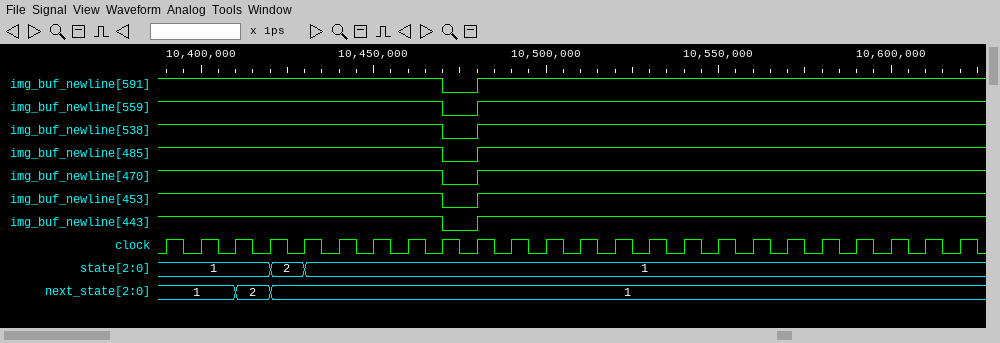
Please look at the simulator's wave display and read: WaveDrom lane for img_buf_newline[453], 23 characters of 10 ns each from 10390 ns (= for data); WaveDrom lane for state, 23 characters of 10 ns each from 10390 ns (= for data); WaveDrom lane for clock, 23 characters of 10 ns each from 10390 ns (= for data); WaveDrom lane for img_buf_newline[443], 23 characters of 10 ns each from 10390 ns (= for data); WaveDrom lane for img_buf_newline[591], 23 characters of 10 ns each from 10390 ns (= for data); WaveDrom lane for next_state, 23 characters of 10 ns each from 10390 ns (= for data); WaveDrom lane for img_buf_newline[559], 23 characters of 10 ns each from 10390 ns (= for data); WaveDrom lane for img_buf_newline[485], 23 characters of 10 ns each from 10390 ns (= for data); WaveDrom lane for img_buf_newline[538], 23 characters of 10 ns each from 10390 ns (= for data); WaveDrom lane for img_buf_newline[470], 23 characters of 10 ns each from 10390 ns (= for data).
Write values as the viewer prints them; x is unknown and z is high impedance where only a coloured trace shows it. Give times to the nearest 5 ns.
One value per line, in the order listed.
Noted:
{name: 'img_buf_newline[453]', wave: '1.......01.............'}
{name: 'state', wave: '=..==..................', data: '1 2 1'}
{name: 'clock', wave: 'p......................'}
{name: 'img_buf_newline[443]', wave: '1.......01.............'}
{name: 'img_buf_newline[591]', wave: '1.......01.............'}
{name: 'next_state', wave: '=.==...................', data: '1 2 1'}
{name: 'img_buf_newline[559]', wave: '1.......01.............'}
{name: 'img_buf_newline[485]', wave: '1.......01.............'}
{name: 'img_buf_newline[538]', wave: '1.......01.............'}
{name: 'img_buf_newline[470]', wave: '1.......01.............'}
